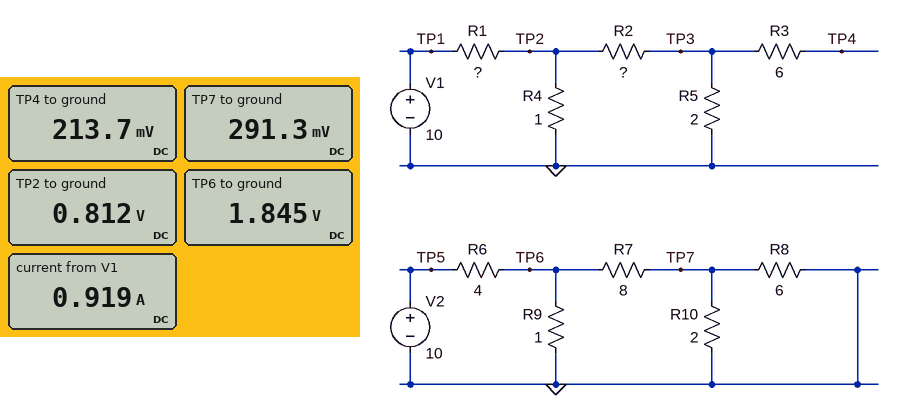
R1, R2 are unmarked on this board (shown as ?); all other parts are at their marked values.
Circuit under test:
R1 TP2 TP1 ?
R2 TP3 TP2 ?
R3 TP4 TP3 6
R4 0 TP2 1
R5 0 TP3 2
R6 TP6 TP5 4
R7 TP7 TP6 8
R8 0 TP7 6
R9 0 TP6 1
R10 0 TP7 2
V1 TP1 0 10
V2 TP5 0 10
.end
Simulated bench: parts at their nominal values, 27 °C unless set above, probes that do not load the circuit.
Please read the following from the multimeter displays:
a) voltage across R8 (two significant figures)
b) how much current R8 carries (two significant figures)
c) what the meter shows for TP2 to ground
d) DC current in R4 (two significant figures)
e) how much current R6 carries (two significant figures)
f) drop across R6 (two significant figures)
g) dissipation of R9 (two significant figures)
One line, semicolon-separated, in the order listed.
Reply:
290 mV; 49 mA; 0.812 V; 810 mA; 2.0 A; 8.2 V; 3.4 W
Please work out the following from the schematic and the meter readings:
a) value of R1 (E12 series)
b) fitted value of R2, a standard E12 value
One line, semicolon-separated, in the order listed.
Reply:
10 Ω; 5.6 Ω
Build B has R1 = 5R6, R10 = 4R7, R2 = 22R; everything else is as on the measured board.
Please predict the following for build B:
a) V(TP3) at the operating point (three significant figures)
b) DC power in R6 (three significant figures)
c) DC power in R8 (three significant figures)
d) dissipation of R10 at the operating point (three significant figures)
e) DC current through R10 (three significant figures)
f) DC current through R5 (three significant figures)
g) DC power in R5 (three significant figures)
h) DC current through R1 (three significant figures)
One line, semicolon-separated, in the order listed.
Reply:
122 mV; 16.6 W; 35.4 mW; 45.2 mW; 98.1 mA; 61.0 mA; 7.44 mW; 1.52 A
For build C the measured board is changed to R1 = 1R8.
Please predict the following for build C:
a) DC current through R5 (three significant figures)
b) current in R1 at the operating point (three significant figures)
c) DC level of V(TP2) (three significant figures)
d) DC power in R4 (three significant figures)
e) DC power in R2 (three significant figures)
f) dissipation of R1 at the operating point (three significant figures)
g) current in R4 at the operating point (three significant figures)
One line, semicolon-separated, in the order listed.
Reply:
433 mA; 3.73 A; 3.29 V; 10.8 W; 1.05 W; 25.0 W; 3.29 A
